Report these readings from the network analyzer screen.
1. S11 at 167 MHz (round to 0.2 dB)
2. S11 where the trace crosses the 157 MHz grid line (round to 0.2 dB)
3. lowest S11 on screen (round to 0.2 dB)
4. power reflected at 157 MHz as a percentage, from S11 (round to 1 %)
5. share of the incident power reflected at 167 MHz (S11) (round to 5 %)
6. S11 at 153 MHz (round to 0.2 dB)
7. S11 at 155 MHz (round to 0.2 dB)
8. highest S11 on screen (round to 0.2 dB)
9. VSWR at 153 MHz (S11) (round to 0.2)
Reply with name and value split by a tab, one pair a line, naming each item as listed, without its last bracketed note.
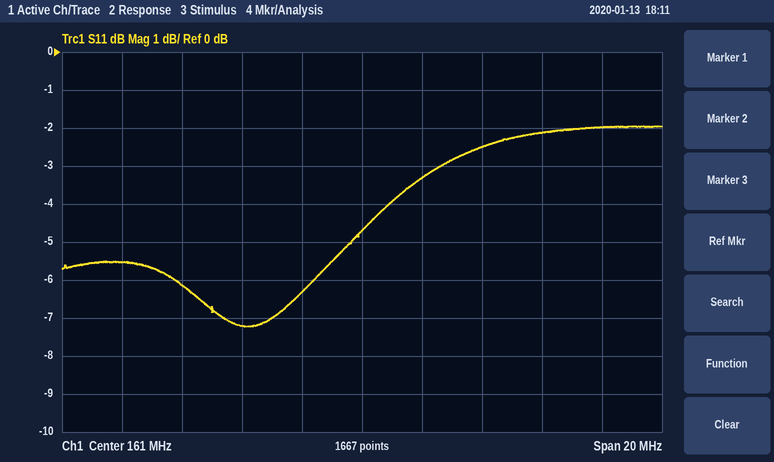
S11 at 167 MHz	-2.2 dB
S11 where the trace crosses the 157 MHz grid line	-7.2 dB
lowest S11 on screen	-7.2 dB
power reflected at 157 MHz as a percentage, from S11	19 %
share of the incident power reflected at 167 MHz (S11)	60 %
S11 at 153 MHz	-5.6 dB
S11 at 155 MHz	-6.2 dB
highest S11 on screen	-2.0 dB
VSWR at 153 MHz (S11)	3.2
